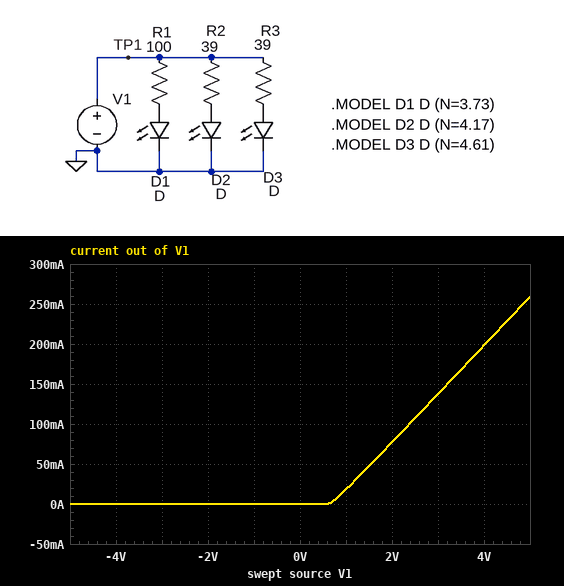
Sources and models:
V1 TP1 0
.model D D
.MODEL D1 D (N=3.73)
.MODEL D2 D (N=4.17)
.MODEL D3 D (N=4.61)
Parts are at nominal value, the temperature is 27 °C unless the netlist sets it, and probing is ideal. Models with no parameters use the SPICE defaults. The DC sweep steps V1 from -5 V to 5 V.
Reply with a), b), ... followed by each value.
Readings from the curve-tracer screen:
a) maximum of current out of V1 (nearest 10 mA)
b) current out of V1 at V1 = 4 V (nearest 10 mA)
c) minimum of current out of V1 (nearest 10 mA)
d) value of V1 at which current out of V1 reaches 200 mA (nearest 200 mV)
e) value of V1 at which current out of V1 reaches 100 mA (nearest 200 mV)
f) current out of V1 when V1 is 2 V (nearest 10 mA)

a) 260 mA
b) 200 mA
c) 0 A
d) 4.0 V
e) 2.4 V
f) 80 mA
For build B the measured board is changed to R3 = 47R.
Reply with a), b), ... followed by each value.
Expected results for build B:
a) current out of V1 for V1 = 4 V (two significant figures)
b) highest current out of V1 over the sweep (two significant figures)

a) 180 mA
b) 240 mA
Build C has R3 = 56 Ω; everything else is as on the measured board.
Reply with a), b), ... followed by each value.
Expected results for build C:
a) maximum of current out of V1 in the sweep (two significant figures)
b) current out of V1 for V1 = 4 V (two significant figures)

a) 230 mA
b) 170 mA
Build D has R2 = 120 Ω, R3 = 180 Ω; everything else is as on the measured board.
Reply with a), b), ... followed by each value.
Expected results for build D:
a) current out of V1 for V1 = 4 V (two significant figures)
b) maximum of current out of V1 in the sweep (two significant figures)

a) 78 mA
b) 100 mA
